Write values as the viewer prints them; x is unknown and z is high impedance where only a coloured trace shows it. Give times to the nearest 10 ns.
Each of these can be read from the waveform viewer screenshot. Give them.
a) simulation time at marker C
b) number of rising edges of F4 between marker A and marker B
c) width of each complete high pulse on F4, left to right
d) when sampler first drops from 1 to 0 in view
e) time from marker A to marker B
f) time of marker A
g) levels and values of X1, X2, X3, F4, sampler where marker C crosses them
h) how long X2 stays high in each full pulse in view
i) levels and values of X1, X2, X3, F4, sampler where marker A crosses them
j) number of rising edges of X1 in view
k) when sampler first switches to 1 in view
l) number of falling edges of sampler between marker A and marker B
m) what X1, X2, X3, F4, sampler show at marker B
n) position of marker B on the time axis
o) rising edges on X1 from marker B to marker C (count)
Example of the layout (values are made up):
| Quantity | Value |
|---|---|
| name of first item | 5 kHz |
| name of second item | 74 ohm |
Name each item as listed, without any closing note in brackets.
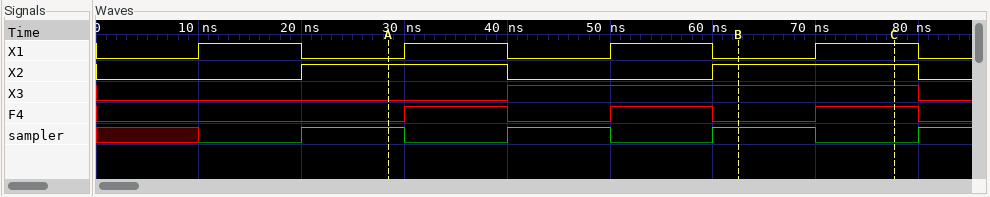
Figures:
| Quantity | Value |
|---|---|
| simulation time at marker C | 80 ns |
| number of rising edges of F4 between marker A and marker B | 2 |
| width of each complete high pulse on F4, left to right | 10 ns, 10 ns, 10 ns |
| when sampler first drops from 1 to 0 in view | 30 ns |
| time from marker A to marker B | 30 ns |
| time of marker A | 30 ns |
| levels and values of X1, X2, X3, F4, sampler where marker C crosses them | X1=1, X2=1, X3=1, F4=1, sampler=0 |
| how long X2 stays high in each full pulse in view | 20 ns, 20 ns |
| levels and values of X1, X2, X3, F4, sampler where marker A crosses them | X1=0, X2=1, X3=0, F4=0, sampler=1 |
| number of rising edges of X1 in view | 4 |
| when sampler first switches to 1 in view | 20 ns |
| number of falling edges of sampler between marker A and marker B | 2 |
| what X1, X2, X3, F4, sampler show at marker B | X1=0, X2=1, X3=1, F4=0, sampler=1 |
| position of marker B on the time axis | 60 ns |
| rising edges on X1 from marker B to marker C | 1 |
